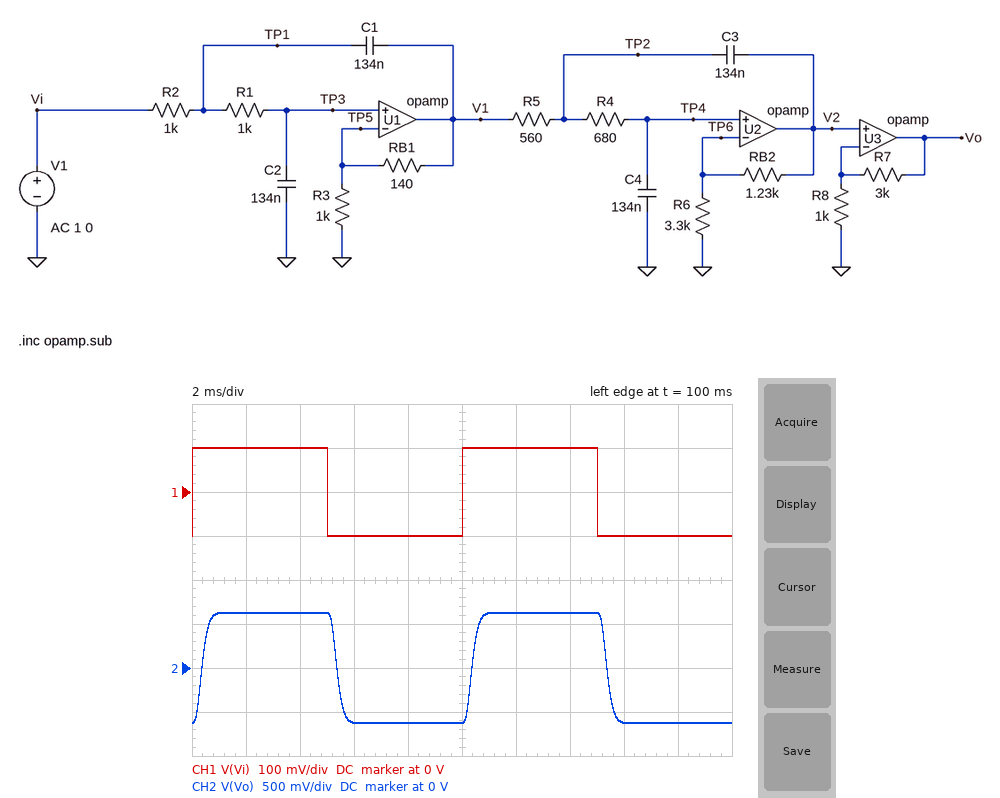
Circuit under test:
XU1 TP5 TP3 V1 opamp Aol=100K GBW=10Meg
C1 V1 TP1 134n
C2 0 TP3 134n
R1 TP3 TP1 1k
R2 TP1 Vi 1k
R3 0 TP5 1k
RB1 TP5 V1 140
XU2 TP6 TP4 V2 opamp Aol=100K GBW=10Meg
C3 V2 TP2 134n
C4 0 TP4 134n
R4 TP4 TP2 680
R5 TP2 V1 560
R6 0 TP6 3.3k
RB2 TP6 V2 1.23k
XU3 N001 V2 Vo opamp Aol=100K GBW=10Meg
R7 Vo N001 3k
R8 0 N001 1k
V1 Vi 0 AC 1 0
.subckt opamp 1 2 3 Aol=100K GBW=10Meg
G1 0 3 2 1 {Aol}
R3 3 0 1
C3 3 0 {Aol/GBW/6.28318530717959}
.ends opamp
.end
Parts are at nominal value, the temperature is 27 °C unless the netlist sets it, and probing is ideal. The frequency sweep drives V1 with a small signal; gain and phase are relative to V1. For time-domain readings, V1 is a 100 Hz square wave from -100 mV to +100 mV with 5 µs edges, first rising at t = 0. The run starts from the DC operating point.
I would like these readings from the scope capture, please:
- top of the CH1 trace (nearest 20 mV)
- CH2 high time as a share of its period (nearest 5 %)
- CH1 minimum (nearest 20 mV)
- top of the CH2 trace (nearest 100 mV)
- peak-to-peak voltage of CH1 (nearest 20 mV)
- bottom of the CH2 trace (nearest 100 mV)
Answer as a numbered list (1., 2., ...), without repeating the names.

1. 100 mV
2. 50 %
3. -100 mV
4. 600 mV
5. 200 mV
6. -600 mV
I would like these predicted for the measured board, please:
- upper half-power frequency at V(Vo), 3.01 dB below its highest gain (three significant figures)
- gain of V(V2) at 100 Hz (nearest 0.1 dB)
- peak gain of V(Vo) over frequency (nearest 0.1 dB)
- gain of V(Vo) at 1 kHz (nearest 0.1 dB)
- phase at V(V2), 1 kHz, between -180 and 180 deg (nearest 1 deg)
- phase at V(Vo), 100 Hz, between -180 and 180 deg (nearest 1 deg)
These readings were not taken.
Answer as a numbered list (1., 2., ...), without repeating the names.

1. 753 Hz
2. 3.8 dB
3. 15.9 dB
4. 10.8 dB
5. -129 deg
6. -14 deg
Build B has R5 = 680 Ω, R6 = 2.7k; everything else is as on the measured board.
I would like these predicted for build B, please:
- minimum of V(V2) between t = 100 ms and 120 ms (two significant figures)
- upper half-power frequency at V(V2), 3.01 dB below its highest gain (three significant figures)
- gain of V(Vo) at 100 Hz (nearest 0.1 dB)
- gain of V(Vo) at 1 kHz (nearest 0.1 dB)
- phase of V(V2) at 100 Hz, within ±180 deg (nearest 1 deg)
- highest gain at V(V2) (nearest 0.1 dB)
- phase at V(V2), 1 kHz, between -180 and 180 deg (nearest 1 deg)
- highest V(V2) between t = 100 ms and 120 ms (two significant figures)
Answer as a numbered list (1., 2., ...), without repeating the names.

1. -170 mV
2. 772 Hz
3. 16.4 dB
4. 11.5 dB
5. -14 deg
6. 4.4 dB
7. -132 deg
8. 170 mV
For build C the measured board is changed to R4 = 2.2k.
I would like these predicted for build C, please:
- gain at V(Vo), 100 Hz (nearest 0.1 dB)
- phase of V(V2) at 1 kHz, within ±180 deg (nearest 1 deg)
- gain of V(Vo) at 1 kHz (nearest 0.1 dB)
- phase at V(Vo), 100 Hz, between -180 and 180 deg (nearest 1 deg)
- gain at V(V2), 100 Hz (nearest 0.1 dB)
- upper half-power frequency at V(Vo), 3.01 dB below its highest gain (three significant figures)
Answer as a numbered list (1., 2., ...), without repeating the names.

1. 15.8 dB
2. -166 deg
3. 5.2 dB
4. -21 deg
5. 3.7 dB
6. 453 Hz
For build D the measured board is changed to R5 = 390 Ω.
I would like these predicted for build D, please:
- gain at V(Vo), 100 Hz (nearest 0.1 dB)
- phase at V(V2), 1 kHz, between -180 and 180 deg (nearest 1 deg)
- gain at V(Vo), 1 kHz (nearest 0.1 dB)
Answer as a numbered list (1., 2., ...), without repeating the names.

1. 15.9 dB
2. -123 deg
3. 10.9 dB
